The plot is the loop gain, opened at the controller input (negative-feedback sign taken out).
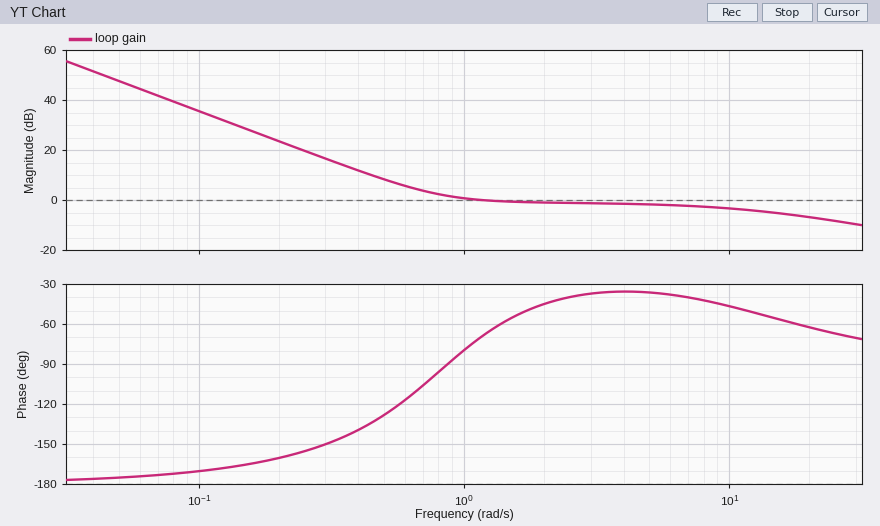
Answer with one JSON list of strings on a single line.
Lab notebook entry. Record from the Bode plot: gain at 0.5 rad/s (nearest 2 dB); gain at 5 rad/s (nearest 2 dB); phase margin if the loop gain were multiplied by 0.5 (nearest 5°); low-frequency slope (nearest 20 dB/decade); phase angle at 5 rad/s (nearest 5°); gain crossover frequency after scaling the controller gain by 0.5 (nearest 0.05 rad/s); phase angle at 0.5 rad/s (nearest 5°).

["8 dB", "-2 dB", "60°", "-40 dB/decade", "-35°", "0.60 rad/s", "-130°"]
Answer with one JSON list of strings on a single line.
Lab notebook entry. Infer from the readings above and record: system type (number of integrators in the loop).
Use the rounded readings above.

["2"]
